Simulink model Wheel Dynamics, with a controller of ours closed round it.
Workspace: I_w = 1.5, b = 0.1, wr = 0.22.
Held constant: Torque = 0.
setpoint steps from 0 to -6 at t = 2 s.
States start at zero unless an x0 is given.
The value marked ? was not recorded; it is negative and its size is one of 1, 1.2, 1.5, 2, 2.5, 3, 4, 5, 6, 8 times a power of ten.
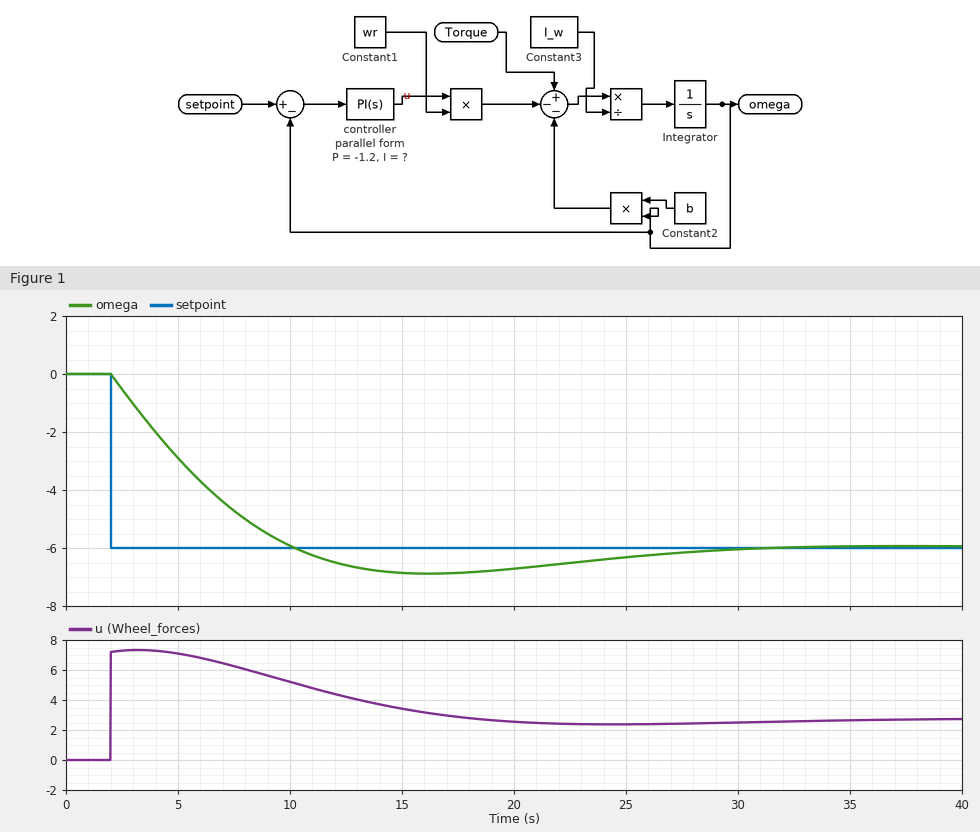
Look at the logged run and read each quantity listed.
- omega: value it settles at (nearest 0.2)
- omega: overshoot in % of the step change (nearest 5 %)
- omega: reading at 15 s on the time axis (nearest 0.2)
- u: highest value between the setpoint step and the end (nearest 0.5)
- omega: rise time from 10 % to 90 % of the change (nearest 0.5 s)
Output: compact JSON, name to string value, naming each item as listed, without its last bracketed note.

{"omega: value it settles at": "-6.0", "omega: overshoot in % of the step change": "15 %", "omega: reading at 15 s on the time axis": "-6.8", "u: highest value between the setpoint step and the end": "7.5", "omega: rise time from 10 % to 90 % of the change": "6.0 s"}
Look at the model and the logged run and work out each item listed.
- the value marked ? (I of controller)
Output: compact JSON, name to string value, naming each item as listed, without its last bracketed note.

{"the value marked ?": "-0.25"}
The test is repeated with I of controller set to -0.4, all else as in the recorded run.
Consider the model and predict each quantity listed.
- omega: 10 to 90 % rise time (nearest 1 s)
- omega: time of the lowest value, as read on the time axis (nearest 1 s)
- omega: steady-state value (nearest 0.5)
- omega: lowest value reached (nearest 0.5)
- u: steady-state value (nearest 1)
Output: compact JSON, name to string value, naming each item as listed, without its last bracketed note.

{"omega: 10 to 90 % rise time": "5 s", "omega: time of the lowest value, as read on the time axis": "13 s", "omega: steady-state value": "-6.0", "omega: lowest value reached": "-7.5", "u: steady-state value": "3"}
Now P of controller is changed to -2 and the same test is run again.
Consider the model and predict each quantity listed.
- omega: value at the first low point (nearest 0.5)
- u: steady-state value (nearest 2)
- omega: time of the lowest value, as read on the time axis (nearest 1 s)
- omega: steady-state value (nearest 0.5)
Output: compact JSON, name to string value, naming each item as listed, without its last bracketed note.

{"omega: value at the first low point": "-6.5", "u: steady-state value": "2", "omega: time of the lowest value, as read on the time axis": "15 s", "omega: steady-state value": "-6.0"}
